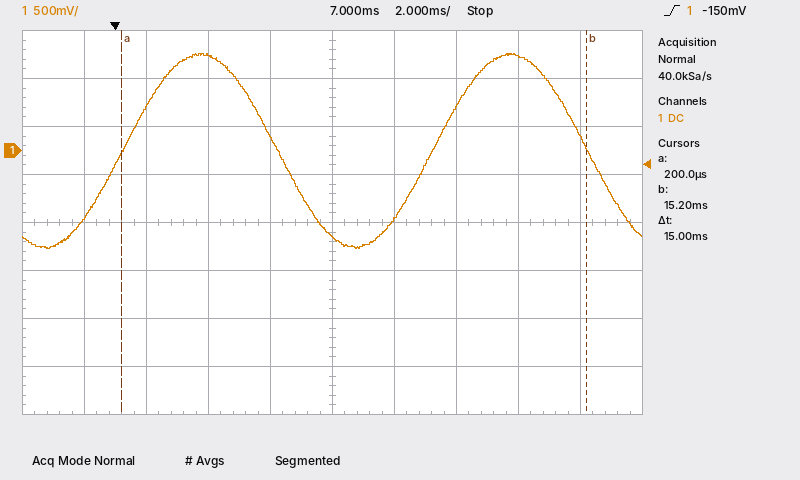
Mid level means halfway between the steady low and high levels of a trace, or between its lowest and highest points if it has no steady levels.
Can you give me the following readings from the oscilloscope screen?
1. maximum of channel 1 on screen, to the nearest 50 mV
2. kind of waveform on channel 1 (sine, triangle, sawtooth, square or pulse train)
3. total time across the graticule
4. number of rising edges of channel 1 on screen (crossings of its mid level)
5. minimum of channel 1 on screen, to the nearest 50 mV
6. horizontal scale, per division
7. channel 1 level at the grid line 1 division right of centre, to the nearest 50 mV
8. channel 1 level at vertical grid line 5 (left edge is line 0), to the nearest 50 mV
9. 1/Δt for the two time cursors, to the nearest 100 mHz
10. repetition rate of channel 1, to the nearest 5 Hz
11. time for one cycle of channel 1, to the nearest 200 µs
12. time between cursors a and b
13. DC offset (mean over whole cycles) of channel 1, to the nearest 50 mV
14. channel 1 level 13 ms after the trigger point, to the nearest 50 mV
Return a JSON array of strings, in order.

["1.00 V", "sine", "20 ms", "2", "-1.00 V", "2 ms", "-700 mV", "-900 mV", "66.7 Hz", "100 Hz", "10.0 ms", "15 ms", "0 mV", "1.00 V"]
